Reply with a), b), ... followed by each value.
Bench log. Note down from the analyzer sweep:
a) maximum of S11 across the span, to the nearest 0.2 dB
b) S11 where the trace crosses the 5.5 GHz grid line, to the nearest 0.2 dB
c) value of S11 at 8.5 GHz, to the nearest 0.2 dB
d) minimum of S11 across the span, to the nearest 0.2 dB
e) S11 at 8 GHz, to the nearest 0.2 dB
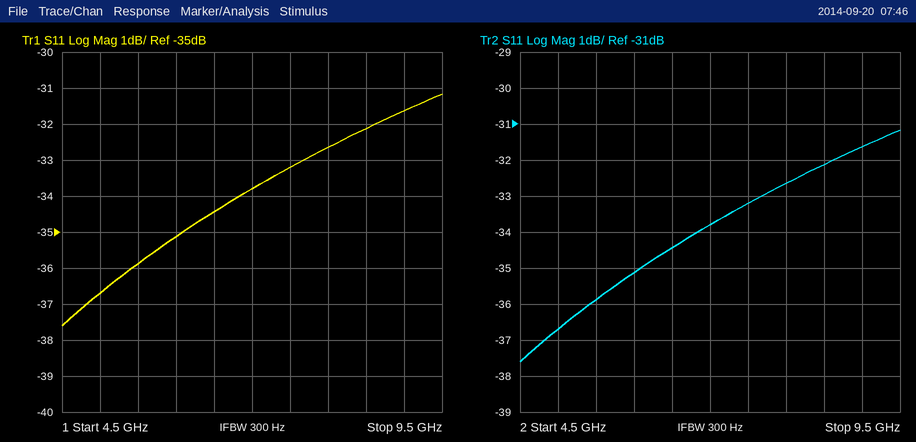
a) -31.2 dB
b) -35.8 dB
c) -32.2 dB
d) -37.6 dB
e) -32.6 dB
